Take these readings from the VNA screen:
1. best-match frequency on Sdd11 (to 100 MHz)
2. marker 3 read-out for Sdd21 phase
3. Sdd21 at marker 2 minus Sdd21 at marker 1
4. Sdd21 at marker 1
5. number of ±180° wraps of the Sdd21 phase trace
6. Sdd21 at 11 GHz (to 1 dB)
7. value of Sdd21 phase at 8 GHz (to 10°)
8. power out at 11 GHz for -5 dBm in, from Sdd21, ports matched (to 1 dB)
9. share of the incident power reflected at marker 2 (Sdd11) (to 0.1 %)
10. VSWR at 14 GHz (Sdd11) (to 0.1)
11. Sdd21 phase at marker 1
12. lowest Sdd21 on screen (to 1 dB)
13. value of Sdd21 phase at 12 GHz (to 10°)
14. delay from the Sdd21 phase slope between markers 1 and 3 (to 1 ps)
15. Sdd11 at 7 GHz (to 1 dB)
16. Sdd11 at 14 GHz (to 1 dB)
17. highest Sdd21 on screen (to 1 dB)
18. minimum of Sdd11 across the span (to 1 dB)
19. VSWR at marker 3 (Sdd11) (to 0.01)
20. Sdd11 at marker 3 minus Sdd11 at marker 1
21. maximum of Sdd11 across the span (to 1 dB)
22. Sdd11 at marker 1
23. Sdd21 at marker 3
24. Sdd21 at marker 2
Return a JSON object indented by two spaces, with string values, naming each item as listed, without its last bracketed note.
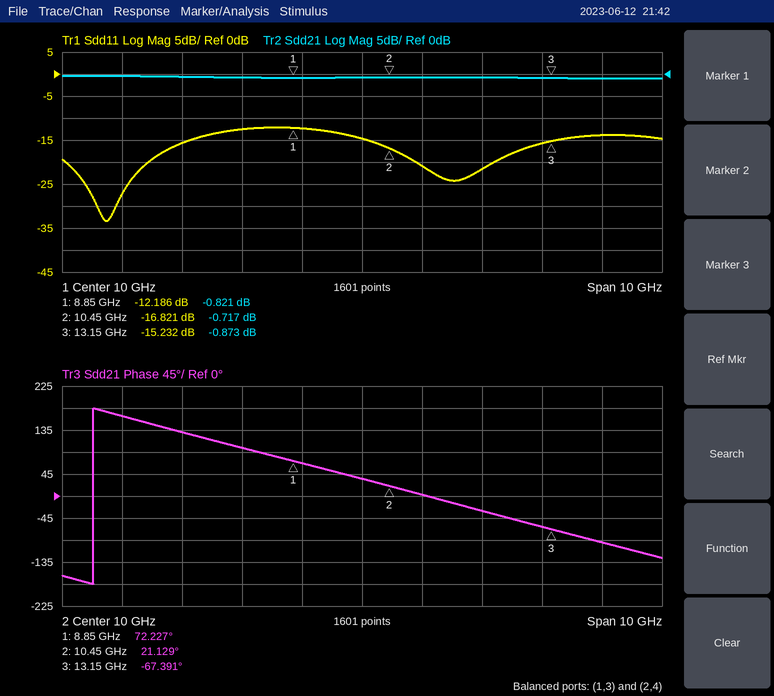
{
  "best-match frequency on Sdd11": "5.7 GHz",
  "marker 3 read-out for Sdd21 phase": "-67.391°",
  "Sdd21 at marker 2 minus Sdd21 at marker 1": "0.104 dB",
  "Sdd21 at marker 1": "-0.821 dB",
  "number of ±180° wraps of the Sdd21 phase trace": "1",
  "Sdd21 at 11 GHz": "-1 dB",
  "value of Sdd21 phase at 8 GHz": "100°",
  "power out at 11 GHz for -5 dBm in, from Sdd21, ports matched": "-6 dBm",
  "share of the incident power reflected at marker 2 (Sdd11)": "2.1 %",
  "VSWR at 14 GHz (Sdd11)": "1.5",
  "Sdd21 phase at marker 1": "72.227°",
  "lowest Sdd21 on screen": "-1 dB",
  "value of Sdd21 phase at 12 GHz": "-30°",
  "delay from the Sdd21 phase slope between markers 1 and 3": "90 ps",
  "Sdd11 at 7 GHz": "-16 dB",
  "Sdd11 at 14 GHz": "-14 dB",
  "highest Sdd21 on screen": "0 dB",
  "minimum of Sdd11 across the span": "-33 dB",
  "VSWR at marker 3 (Sdd11)": "1.42",
  "Sdd11 at marker 3 minus Sdd11 at marker 1": "-3.046 dB",
  "maximum of Sdd11 across the span": "-12 dB",
  "Sdd11 at marker 1": "-12.186 dB",
  "Sdd21 at marker 3": "-0.873 dB",
  "Sdd21 at marker 2": "-0.717 dB"
}
